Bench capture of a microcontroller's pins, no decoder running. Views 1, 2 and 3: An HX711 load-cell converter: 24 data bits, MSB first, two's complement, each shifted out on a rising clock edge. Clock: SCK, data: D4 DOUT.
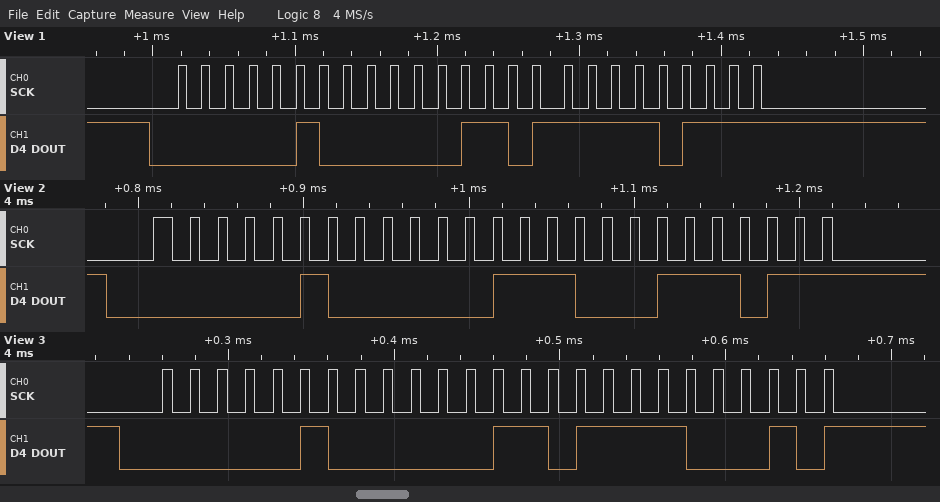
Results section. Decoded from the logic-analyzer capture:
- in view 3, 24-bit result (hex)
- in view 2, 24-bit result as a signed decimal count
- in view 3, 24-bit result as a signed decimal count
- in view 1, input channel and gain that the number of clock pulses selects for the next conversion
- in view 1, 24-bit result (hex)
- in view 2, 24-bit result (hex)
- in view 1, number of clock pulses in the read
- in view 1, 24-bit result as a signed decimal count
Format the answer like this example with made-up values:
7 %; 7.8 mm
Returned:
0x040DE2; 265787; 265698; channel A, gain 128; 0x040DF7; 0x040E3B; 25; 265719
